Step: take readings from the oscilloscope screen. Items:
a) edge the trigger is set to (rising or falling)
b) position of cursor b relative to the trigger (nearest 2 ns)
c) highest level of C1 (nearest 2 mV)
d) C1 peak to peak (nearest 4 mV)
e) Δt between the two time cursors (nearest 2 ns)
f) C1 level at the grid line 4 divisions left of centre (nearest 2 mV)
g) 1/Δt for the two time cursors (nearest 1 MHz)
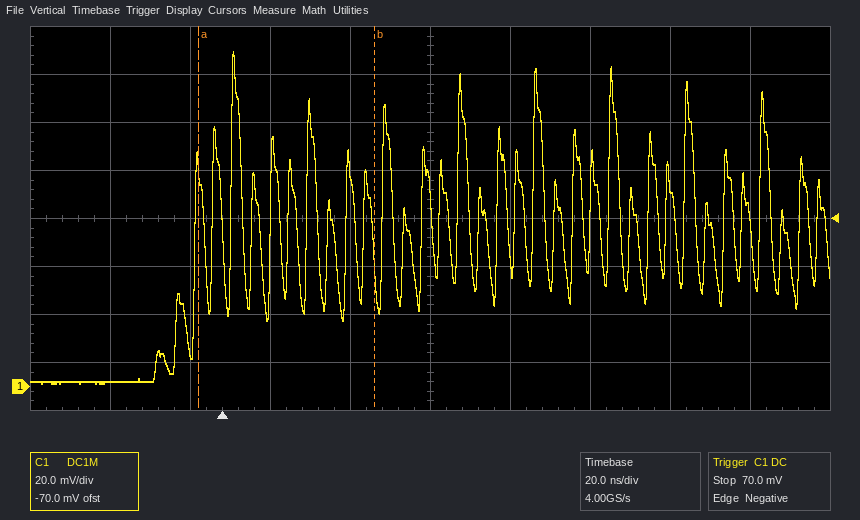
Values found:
falling
+38 ns
140 mV
140 mV
44 ns
2 mV
23 MHz
